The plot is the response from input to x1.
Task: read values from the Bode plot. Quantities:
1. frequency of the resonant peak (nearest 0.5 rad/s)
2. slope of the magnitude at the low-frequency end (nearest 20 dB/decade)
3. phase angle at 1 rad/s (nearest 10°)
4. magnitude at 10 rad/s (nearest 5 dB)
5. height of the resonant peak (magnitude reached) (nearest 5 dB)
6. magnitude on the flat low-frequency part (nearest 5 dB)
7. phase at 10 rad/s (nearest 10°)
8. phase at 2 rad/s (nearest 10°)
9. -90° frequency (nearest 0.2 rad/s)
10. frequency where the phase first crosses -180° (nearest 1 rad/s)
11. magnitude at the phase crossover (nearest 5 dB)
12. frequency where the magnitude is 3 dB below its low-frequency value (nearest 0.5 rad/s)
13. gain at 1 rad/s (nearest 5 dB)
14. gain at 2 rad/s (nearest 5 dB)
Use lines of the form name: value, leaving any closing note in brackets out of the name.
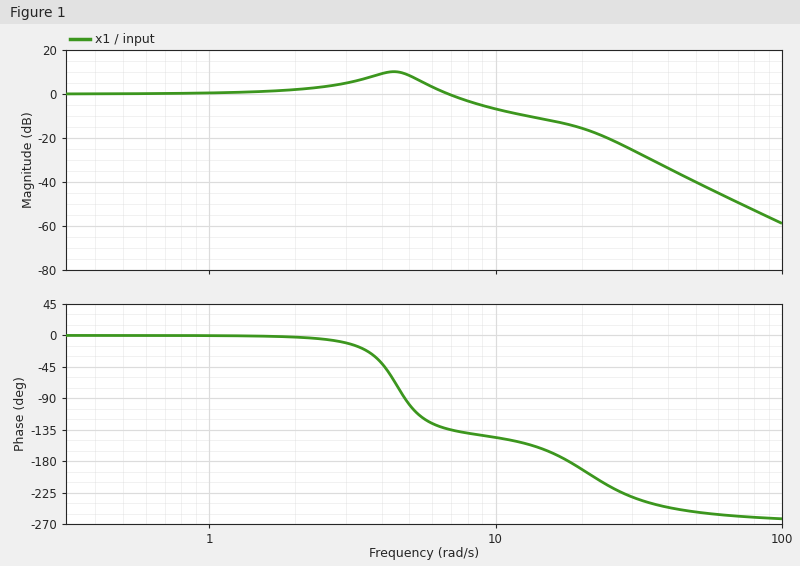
frequency of the resonant peak: 4.5 rad/s
slope of the magnitude at the low-frequency end: 0 dB/decade
phase angle at 1 rad/s: 0°
magnitude at 10 rad/s: -5 dB
height of the resonant peak (magnitude reached): 10 dB
magnitude on the flat low-frequency part: 0 dB
phase at 10 rad/s: -150°
phase at 2 rad/s: 0°
-90° frequency: 4.8 rad/s
frequency where the phase first crosses -180°: 18 rad/s
magnitude at the phase crossover: -15 dB
frequency where the magnitude is 3 dB below its low-frequency value: 8.0 rad/s
gain at 1 rad/s: 0 dB
gain at 2 rad/s: 0 dB
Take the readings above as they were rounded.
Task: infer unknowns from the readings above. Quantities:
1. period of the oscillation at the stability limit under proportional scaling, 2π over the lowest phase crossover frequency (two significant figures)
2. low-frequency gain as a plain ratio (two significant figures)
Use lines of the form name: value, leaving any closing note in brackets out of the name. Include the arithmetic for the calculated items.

period of the oscillation at the stability limit under proportional scaling, 2π over the lowest phase crossover frequency: 2π / 18 = 0.35 s
low-frequency gain as a plain ratio: 10^(0 / 20) = 1.0
